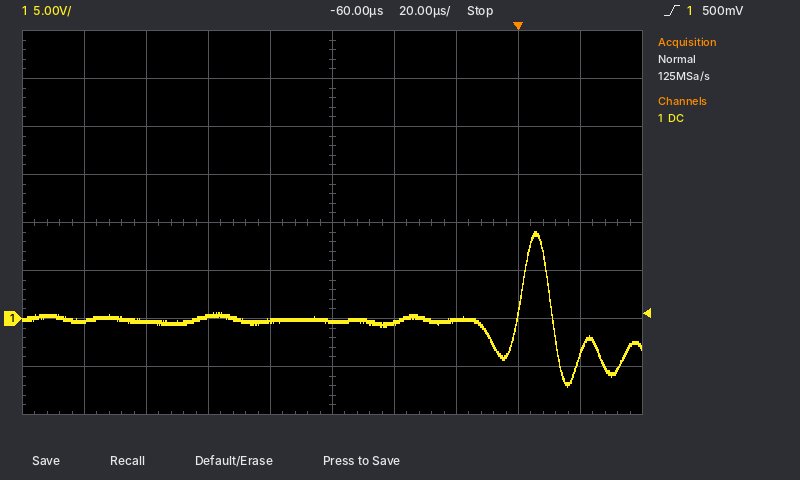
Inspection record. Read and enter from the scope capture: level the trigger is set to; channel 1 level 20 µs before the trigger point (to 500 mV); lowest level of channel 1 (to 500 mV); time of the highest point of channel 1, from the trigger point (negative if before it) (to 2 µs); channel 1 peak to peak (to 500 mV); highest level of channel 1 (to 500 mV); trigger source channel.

500 mV
0.0 V
-7.0 V
+6 µs
16.0 V
9.0 V
channel 1
